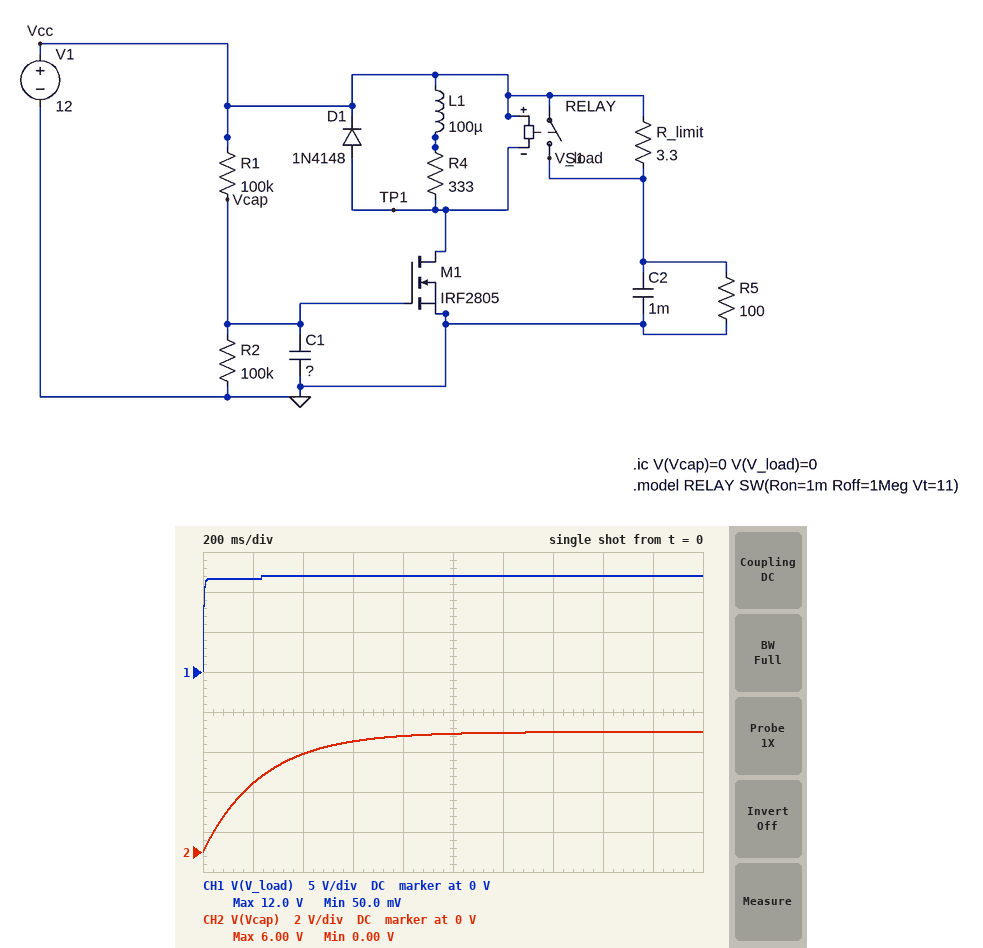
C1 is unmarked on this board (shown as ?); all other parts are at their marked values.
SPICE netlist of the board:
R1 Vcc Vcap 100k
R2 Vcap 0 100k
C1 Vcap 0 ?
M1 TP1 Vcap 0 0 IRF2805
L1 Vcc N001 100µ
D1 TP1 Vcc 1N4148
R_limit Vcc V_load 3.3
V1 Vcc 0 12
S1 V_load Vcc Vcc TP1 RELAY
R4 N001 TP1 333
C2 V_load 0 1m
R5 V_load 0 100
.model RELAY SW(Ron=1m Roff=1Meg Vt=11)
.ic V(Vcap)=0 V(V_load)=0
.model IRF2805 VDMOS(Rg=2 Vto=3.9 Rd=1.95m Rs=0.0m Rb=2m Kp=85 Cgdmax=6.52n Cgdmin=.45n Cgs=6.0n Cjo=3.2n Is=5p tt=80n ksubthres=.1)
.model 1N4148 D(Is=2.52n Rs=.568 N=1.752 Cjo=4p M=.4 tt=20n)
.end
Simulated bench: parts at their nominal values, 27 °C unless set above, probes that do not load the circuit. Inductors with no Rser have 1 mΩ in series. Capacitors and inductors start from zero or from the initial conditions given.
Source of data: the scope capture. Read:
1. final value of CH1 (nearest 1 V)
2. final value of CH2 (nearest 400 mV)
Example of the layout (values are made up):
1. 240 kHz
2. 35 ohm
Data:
1. 12 V
2. 6.0 V
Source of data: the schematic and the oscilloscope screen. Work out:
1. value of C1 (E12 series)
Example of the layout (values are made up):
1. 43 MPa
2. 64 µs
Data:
1. 4.7 µF
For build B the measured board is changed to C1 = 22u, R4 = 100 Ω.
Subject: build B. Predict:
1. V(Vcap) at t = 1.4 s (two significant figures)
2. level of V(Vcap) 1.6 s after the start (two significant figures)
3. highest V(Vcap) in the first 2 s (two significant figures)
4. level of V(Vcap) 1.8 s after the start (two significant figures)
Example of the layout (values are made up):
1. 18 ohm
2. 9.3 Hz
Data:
1. 4.3 V
2. 4.6 V
3. 5.0 V
4. 4.8 V
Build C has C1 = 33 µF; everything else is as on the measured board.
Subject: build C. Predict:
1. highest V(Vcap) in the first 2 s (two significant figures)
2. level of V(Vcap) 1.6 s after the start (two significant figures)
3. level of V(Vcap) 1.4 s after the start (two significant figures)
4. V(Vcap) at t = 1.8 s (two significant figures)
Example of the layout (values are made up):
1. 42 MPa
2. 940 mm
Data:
1. 4.2 V
2. 3.7 V
3. 3.4 V
4. 4.0 V
